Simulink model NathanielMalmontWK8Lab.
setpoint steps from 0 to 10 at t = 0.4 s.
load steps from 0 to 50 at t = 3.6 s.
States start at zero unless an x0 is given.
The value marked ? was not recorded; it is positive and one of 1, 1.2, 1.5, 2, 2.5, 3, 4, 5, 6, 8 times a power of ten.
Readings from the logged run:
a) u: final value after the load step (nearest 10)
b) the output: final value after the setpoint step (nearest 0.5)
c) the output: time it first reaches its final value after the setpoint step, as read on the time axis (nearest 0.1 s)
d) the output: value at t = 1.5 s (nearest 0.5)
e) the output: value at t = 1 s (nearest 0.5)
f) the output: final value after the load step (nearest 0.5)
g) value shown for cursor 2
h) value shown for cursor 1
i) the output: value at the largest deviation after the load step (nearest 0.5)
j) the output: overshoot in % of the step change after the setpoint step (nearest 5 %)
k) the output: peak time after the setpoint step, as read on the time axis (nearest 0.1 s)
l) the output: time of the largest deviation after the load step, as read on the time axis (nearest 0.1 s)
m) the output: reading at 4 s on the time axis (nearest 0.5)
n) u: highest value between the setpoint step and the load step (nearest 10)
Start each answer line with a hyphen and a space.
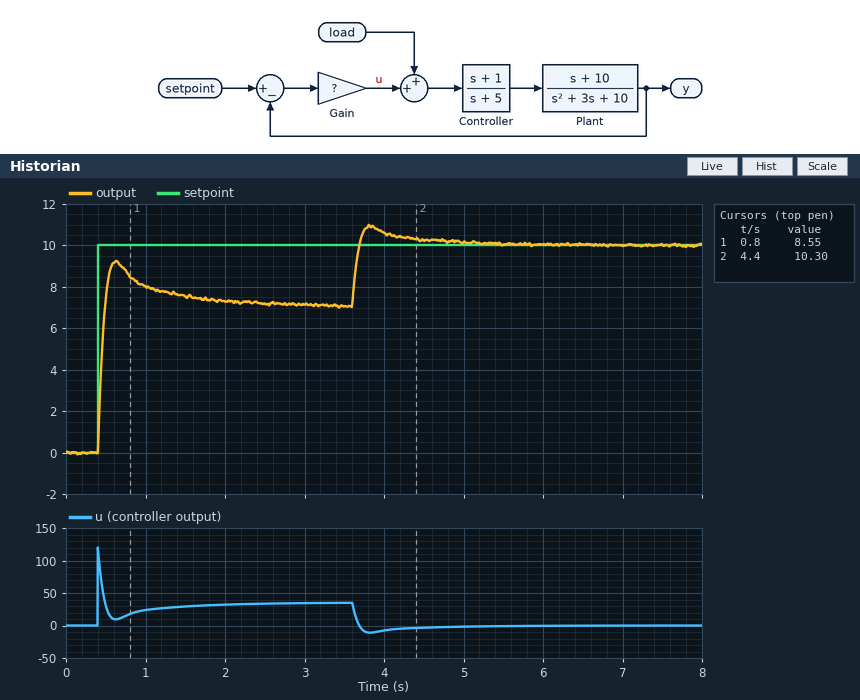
- 0
- 7.0
- 0.5 s
- 7.5
- 8.0
- 10.0
- 10.30
- 8.55
- 11.0
- 30 %
- 0.6 s
- 3.8 s
- 10.5
- 120
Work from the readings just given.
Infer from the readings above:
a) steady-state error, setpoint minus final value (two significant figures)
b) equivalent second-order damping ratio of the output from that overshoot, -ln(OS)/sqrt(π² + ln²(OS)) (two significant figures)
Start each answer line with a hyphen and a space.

- 3.0
- 0.36
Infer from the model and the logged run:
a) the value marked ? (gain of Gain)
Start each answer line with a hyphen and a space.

- 12
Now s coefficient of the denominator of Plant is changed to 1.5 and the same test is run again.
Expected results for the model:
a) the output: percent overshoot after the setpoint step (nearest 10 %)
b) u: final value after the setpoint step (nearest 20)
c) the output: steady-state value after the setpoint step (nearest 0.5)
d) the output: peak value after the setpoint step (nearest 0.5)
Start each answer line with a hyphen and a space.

- 40 %
- 40
- 7.0
- 10.0
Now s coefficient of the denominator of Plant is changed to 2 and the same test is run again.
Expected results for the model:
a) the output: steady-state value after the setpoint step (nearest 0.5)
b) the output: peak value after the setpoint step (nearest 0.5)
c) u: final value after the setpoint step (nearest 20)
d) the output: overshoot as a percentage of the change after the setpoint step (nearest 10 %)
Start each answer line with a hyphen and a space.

- 7.0
- 9.5
- 40
- 40 %
